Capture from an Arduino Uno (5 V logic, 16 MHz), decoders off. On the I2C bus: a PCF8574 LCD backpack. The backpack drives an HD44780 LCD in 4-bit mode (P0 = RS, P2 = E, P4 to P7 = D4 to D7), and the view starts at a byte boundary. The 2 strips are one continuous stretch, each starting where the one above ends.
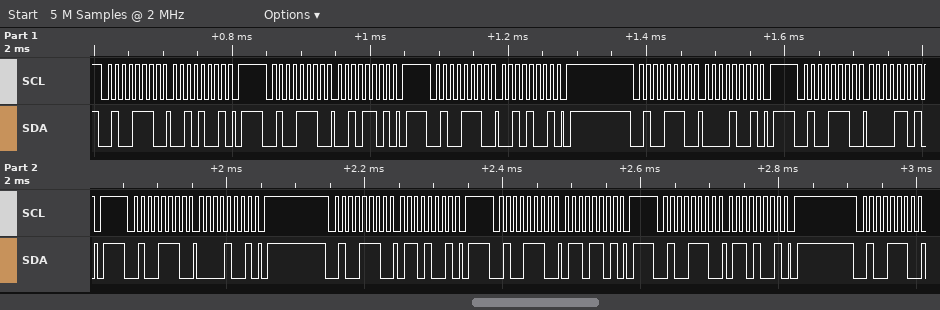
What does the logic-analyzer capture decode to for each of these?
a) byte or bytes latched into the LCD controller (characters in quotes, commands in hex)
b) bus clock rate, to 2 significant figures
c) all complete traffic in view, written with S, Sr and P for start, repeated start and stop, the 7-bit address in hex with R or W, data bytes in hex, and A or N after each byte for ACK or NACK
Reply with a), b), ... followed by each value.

a) ' '
b) 100 kHz
c) S 27W A 29 A P S 27W A 2D A P S 27W A 29 A P S 27W A 09 A P S 27W A 0D A P S 27W A 09 A P S 27W A 69 A P S 27W A 6D A P S 27W A 69 A P S 27W A
